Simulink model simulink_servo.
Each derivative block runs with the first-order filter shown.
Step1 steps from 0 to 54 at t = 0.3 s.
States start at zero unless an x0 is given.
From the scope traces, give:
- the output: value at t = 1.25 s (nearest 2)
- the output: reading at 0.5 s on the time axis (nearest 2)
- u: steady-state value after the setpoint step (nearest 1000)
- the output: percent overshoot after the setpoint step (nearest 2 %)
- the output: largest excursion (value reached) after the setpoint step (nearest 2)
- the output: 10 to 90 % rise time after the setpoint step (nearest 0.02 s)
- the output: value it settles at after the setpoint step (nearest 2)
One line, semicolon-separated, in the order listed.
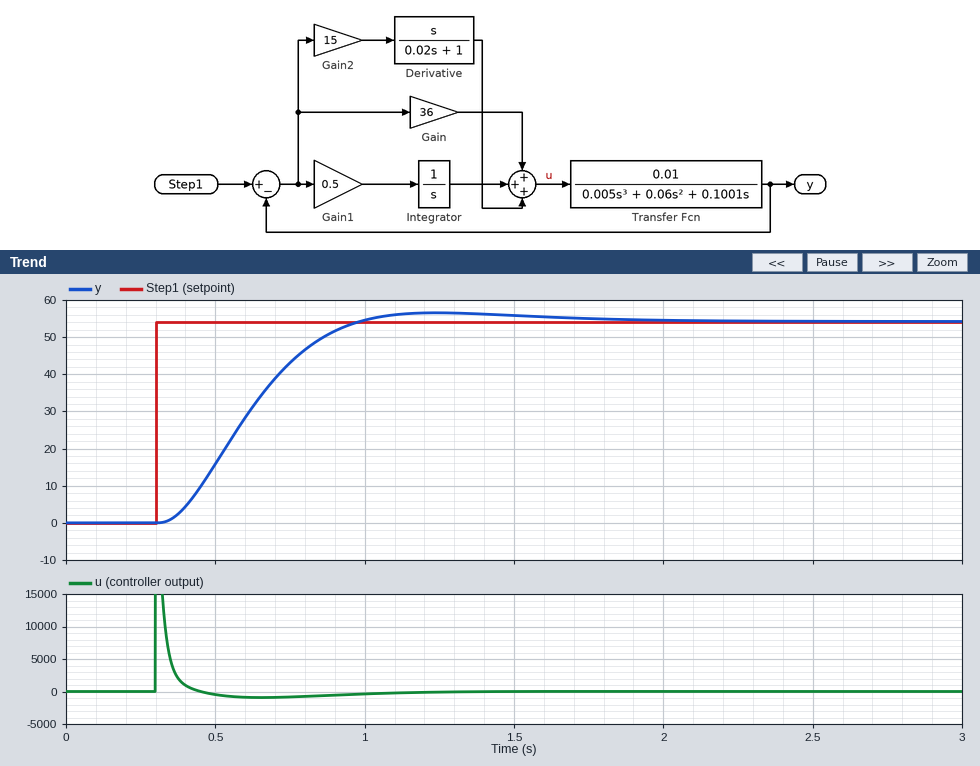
56; 16; 0; 4 %; 56; 0.42 s; 54
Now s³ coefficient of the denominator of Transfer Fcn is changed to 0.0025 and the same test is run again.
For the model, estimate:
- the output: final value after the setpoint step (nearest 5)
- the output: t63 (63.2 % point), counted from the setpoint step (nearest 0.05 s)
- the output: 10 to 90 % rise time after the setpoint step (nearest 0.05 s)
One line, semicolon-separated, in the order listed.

55; 0.35 s; 0.50 s
